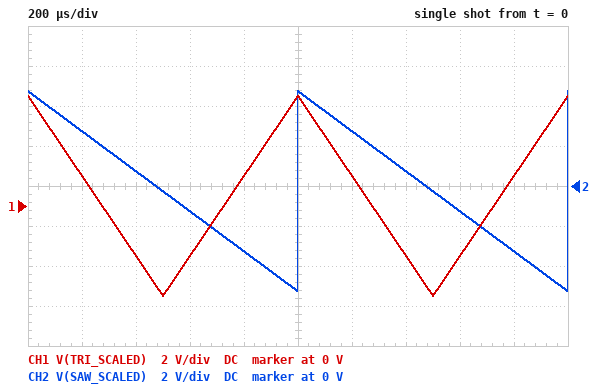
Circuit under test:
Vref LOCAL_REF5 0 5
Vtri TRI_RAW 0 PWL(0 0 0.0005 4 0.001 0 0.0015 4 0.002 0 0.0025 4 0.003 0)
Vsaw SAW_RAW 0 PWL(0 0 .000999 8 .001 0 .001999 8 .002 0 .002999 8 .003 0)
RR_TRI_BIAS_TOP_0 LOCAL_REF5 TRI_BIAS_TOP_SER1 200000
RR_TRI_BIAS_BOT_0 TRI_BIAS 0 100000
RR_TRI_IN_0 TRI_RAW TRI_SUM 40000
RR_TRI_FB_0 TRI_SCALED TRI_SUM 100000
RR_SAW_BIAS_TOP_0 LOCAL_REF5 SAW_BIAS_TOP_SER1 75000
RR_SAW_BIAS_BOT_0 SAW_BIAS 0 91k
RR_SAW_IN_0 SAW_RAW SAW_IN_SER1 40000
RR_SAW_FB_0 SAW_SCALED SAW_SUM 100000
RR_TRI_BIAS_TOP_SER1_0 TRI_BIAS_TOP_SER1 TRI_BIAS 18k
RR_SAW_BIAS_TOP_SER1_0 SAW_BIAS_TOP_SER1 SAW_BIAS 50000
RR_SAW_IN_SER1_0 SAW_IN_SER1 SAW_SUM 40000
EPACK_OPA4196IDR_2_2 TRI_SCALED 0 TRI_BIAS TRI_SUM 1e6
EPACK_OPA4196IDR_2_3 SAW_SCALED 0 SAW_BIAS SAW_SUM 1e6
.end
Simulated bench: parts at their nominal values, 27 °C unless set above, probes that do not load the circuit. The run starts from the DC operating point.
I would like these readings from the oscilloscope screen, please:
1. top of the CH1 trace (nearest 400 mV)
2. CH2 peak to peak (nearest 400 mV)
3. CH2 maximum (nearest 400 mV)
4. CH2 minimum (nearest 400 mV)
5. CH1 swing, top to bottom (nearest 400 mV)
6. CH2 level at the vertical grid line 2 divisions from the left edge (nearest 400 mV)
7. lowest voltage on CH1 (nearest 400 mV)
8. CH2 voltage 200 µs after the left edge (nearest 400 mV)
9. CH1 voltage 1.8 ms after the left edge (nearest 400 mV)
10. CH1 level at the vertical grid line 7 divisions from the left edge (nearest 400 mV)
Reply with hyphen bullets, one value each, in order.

- 5.6 V
- 10.0 V
- 4.8 V
- -5.2 V
- 10.0 V
- 800 mV
- -4.4 V
- 2.8 V
- 1.6 V
- -2.4 V
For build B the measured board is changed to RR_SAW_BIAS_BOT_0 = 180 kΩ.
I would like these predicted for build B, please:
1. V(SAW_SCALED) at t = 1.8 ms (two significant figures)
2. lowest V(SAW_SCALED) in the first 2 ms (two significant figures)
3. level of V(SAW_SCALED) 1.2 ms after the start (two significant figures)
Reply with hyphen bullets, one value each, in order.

- -1.4 V
- -3.4 V
- 4.6 V
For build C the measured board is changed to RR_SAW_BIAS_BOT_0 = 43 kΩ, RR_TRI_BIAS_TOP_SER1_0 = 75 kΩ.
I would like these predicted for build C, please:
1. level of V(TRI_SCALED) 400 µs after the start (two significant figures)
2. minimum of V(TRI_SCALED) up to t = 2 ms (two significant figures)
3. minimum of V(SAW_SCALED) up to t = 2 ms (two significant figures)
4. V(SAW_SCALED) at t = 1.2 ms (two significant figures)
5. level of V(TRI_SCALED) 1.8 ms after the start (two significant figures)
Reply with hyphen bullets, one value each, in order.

- -3.3 V
- -5.3 V
- -7.1 V
- 880 mV
- 670 mV
